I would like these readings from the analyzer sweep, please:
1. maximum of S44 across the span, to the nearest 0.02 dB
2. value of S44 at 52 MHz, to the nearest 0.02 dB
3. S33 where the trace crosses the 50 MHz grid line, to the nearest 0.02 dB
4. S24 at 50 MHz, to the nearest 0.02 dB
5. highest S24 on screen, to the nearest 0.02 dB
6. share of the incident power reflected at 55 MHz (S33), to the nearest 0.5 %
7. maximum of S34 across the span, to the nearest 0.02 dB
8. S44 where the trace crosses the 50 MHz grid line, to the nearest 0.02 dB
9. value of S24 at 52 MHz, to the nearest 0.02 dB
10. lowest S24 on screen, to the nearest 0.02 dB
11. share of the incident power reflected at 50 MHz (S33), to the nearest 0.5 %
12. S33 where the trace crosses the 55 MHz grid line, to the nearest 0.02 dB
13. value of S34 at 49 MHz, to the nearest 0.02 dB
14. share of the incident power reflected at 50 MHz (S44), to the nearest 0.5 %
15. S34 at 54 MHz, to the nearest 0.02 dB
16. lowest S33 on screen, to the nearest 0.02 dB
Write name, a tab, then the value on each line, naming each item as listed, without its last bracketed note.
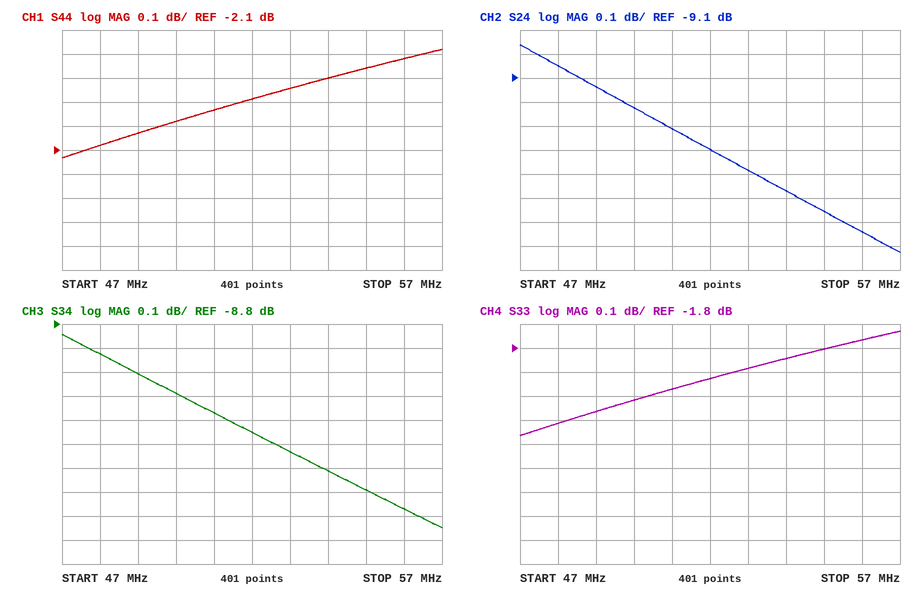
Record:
maximum of S44 across the span, to the nearest 0.02 dB	-1.68 dB
value of S44 at 52 MHz, to the nearest 0.02 dB	-1.88 dB
S33 where the trace crosses the 50 MHz grid line, to the nearest 0.02 dB	-2.02 dB
S24 at 50 MHz, to the nearest 0.02 dB	-9.22 dB
highest S24 on screen, to the nearest 0.02 dB	-8.96 dB
share of the incident power reflected at 55 MHz (S33), to the nearest 0.5 %	66.0 %
maximum of S34 across the span, to the nearest 0.02 dB	-8.84 dB
S44 where the trace crosses the 50 MHz grid line, to the nearest 0.02 dB	-1.98 dB
value of S24 at 52 MHz, to the nearest 0.02 dB	-9.40 dB
lowest S24 on screen, to the nearest 0.02 dB	-9.82 dB
share of the incident power reflected at 50 MHz (S33), to the nearest 0.5 %	63.0 %
S33 where the trace crosses the 55 MHz grid line, to the nearest 0.02 dB	-1.80 dB
value of S34 at 49 MHz, to the nearest 0.02 dB	-9.00 dB
share of the incident power reflected at 50 MHz (S44), to the nearest 0.5 %	63.5 %
S34 at 54 MHz, to the nearest 0.02 dB	-9.42 dB
lowest S33 on screen, to the nearest 0.02 dB	-2.16 dB
